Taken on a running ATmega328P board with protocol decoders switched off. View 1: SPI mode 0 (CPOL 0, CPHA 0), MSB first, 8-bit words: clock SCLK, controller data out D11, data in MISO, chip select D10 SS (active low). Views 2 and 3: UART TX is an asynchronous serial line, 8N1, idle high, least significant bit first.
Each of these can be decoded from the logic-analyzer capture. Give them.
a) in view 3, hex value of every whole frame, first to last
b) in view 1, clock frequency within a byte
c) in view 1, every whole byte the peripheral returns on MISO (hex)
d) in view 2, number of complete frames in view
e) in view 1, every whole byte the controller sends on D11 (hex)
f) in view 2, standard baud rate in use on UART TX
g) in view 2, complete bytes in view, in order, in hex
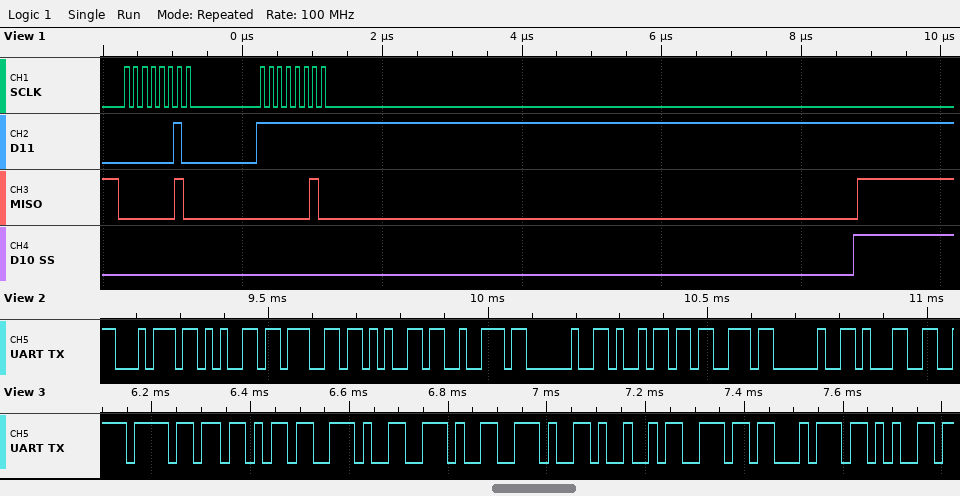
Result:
6F 6B 2E 2E 2E 49 6E 74 65
8 MHz
02 02
10
02 FF
57600 baud
74 65 67 65 72 20 69 73 20 31
